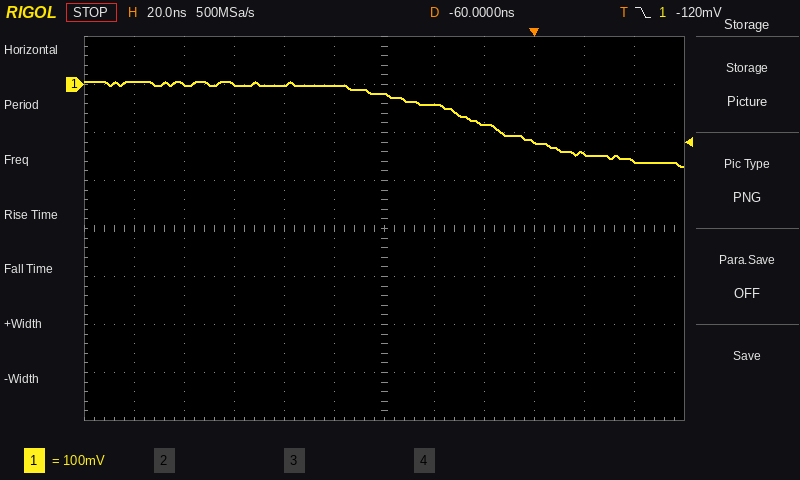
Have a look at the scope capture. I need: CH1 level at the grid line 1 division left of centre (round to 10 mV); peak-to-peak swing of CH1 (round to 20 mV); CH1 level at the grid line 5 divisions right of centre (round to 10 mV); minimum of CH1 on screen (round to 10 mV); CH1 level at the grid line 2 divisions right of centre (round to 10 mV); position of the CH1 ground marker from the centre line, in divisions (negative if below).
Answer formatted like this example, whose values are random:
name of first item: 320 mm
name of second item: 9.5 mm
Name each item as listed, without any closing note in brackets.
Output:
CH1 level at the grid line 1 division left of centre: 0 mV
peak-to-peak swing of CH1: 180 mV
CH1 level at the grid line 5 divisions right of centre: -160 mV
minimum of CH1 on screen: -170 mV
CH1 level at the grid line 2 divisions right of centre: -80 mV
position of the CH1 ground marker from the centre line, in divisions: +3.0 div
